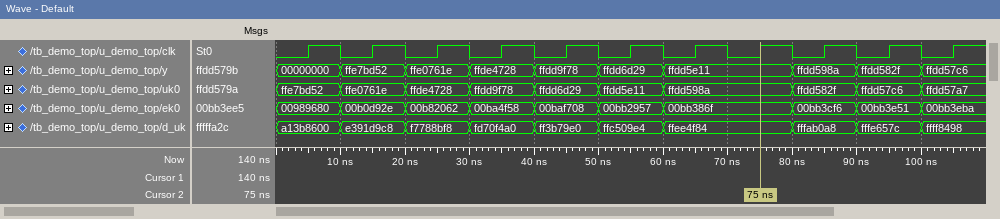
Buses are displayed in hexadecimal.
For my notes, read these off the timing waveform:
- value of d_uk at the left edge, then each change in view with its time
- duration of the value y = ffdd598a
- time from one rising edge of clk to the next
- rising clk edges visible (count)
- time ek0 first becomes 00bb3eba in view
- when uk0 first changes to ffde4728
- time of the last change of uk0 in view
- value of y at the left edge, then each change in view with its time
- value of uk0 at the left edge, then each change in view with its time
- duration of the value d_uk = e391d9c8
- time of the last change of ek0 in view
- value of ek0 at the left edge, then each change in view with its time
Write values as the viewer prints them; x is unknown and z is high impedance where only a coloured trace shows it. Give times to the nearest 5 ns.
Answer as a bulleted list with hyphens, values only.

- a13b8600, e391d9c8 at 10 ns, f7788bf8 at 20 ns, fd70f4a0 at 30 ns, ff3b79e0 at 40 ns, ffc509e4 at 50 ns, ffee4f84 at 60 ns, fffab0a8 at 80 ns, fffe657c at 90 ns, ffff8498 at 100 ns
- 10 ns
- 10 ns
- 11
- 100 ns
- 20 ns
- 100 ns
- 00000000, ffe7bd52 at 10 ns, ffe0761e at 20 ns, ffde4728 at 30 ns, ffdd9f78 at 40 ns, ffdd6d29 at 50 ns, ffdd5e11 at 60 ns, ffdd598a at 80 ns, ffdd582f at 90 ns, ffdd57c6 at 100 ns
- ffe7bd52, ffe0761e at 10 ns, ffde4728 at 20 ns, ffdd9f78 at 30 ns, ffdd6d29 at 40 ns, ffdd5e11 at 50 ns, ffdd598a at 60 ns, ffdd582f at 80 ns, ffdd57c6 at 90 ns, ffdd57a7 at 100 ns
- 10 ns
- 100 ns
- 00989680, 00b0d92e at 10 ns, 00b82062 at 20 ns, 00ba4f58 at 30 ns, 00baf708 at 40 ns, 00bb2957 at 50 ns, 00bb386f at 60 ns, 00bb3cf6 at 80 ns, 00bb3e51 at 90 ns, 00bb3eba at 100 ns
